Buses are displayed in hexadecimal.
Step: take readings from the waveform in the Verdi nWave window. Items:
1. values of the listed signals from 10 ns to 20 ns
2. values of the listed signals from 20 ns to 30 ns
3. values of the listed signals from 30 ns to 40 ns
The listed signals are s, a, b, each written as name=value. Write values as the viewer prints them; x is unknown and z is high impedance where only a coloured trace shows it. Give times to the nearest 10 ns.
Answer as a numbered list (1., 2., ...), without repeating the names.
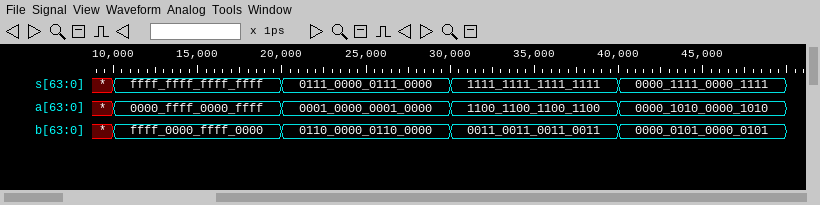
1. s=ffff_ffff_ffff_ffff, a=0000_ffff_0000_ffff, b=ffff_0000_ffff_0000
2. s=0111_0000_0111_0000, a=0001_0000_0001_0000, b=0110_0000_0110_0000
3. s=1111_1111_1111_1111, a=1100_1100_1100_1100, b=0011_0011_0011_0011
